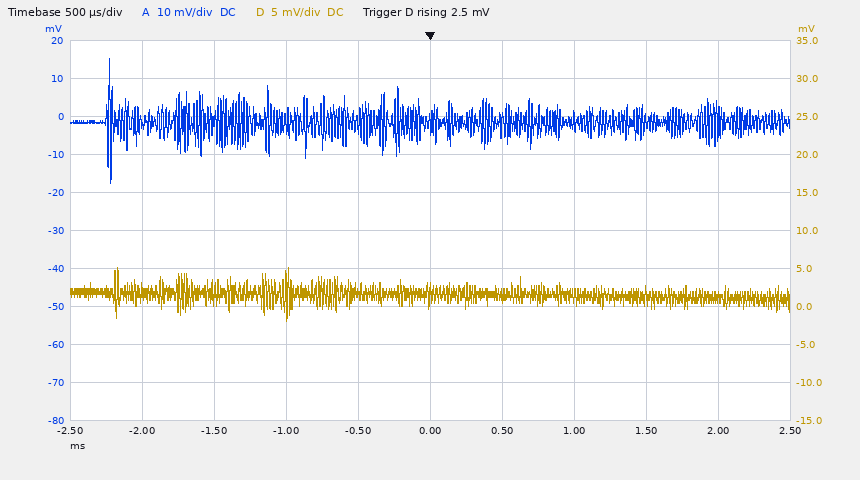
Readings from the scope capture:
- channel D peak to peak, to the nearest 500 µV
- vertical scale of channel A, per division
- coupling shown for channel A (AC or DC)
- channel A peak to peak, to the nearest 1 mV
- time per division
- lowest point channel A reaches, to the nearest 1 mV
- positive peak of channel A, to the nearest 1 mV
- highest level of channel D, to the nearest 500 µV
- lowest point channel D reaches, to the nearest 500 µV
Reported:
7.0 mV
10 mV
DC
33 mV
500 µs
-18 mV
15 mV
5.0 mV
-2.0 mV
